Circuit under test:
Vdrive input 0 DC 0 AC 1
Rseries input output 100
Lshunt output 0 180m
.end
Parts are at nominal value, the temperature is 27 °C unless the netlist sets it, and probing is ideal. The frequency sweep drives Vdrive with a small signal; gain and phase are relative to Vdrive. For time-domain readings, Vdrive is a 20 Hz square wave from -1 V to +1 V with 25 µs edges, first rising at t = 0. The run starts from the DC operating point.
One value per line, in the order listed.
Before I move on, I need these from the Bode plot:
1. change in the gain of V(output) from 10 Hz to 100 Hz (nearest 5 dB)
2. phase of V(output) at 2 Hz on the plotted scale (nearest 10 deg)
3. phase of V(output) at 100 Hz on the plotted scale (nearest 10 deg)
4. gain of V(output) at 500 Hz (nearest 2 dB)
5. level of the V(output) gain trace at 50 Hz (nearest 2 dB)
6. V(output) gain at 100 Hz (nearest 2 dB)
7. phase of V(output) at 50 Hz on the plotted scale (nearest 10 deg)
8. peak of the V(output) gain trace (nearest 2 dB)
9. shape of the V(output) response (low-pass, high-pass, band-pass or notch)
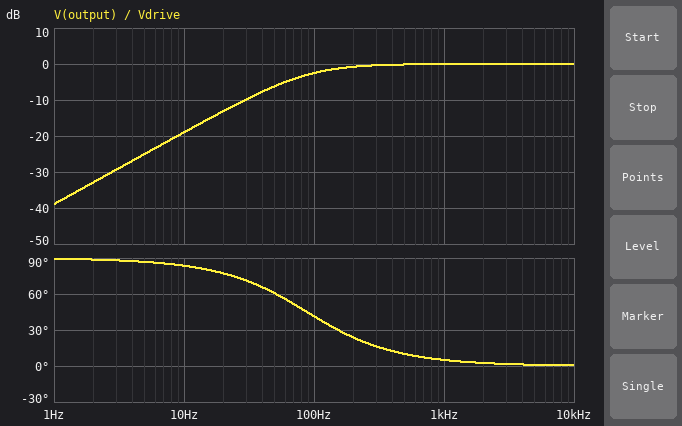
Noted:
15 dB
90 deg
40 deg
0 dB
-6 dB
-2 dB
60 deg
0 dB
high-pass
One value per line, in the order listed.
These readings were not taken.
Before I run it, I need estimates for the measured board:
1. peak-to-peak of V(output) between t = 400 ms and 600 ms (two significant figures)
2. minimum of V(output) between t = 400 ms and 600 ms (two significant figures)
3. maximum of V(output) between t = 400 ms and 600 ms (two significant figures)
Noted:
4.0 V
-2.0 V
2.0 V
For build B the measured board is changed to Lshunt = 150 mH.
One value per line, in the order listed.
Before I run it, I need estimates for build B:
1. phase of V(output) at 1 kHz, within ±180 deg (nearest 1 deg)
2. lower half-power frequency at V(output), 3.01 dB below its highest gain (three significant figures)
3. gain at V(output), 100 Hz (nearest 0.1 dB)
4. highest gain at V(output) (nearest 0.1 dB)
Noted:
6 deg
106 Hz
-3.3 dB
0 dB
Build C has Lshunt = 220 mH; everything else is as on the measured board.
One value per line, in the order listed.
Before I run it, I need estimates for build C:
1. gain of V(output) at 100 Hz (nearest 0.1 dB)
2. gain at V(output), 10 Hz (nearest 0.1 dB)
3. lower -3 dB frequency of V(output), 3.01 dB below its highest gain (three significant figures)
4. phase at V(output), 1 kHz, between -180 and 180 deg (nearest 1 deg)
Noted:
-1.8 dB
-17.3 dB
72.3 Hz
4 deg
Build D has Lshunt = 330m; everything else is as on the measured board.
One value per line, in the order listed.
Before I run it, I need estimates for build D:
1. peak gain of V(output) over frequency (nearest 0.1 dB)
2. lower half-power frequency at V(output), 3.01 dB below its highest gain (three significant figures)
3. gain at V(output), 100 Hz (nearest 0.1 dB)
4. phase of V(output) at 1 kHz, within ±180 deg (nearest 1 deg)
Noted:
0 dB
48.2 Hz
-0.9 dB
3 deg
